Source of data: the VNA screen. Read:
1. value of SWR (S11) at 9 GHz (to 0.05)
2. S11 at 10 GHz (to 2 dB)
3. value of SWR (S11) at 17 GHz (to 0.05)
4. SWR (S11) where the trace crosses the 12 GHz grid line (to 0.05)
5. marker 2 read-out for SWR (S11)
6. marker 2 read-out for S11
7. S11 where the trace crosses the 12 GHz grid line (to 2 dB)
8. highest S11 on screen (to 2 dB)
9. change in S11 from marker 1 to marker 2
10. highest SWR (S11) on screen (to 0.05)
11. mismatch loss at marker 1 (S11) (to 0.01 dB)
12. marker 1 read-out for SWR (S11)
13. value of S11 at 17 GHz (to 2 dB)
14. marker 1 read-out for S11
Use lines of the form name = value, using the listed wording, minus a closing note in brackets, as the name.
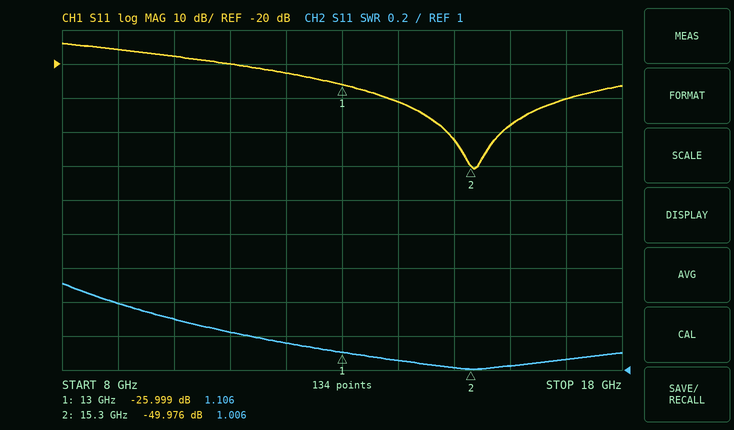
value of SWR (S11) at 9 GHz = 1.40
S11 at 10 GHz = -18 dB
value of SWR (S11) at 17 GHz = 1.05
SWR (S11) where the trace crosses the 12 GHz grid line = 1.15
marker 2 read-out for SWR = 1.006
marker 2 read-out for S11 = -49.976 dB
S11 where the trace crosses the 12 GHz grid line = -22 dB
highest S11 on screen = -14 dB
change in S11 from marker 1 to marker 2 = -23.977 dB
highest SWR (S11) on screen = 1.50
mismatch loss at marker 1 (S11) = 0.01 dB
marker 1 read-out for SWR = 1.106
value of S11 at 17 GHz = -30 dB
marker 1 read-out for S11 = -25.999 dB
